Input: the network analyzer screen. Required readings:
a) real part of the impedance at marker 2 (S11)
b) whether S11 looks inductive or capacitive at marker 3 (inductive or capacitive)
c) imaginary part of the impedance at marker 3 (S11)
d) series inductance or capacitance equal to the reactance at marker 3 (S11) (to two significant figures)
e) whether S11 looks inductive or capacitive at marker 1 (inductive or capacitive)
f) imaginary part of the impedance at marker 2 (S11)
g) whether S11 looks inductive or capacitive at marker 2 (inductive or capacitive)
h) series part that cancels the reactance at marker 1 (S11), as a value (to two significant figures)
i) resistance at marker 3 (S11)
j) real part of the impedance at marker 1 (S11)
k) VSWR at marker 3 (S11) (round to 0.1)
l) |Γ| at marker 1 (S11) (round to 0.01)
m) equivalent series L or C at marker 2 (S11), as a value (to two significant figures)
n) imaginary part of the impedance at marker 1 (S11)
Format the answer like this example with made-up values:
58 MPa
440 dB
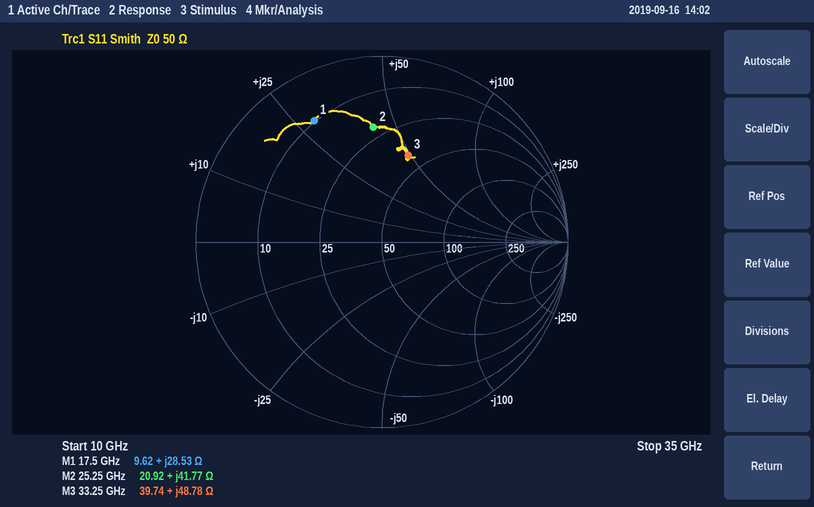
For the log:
20.92 Ω
inductive
+48.78 Ω
230 pH
inductive
+41.77 Ω
inductive
320 fF
39.74 Ω
9.62 Ω
2.9
0.75
260 pH
+28.53 Ω
